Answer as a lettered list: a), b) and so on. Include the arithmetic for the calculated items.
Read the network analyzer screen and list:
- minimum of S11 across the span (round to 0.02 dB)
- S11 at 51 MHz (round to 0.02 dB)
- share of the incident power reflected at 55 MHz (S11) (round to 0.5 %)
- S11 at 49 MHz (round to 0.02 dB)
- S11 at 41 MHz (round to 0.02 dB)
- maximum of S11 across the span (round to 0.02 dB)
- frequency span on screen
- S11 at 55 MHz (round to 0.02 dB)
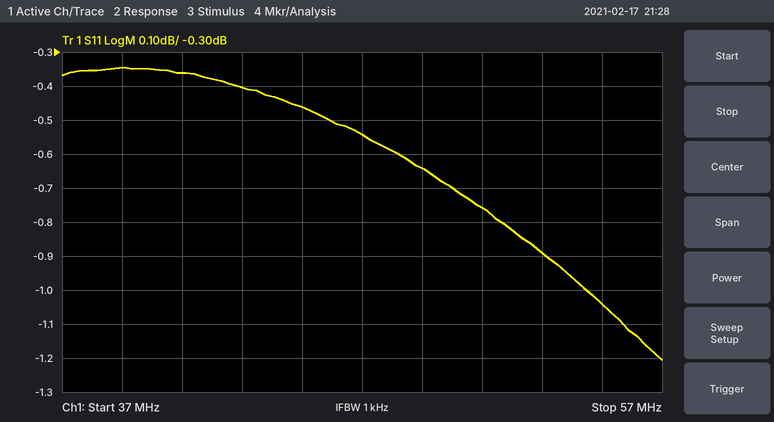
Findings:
a) -1.20 dB
b) -0.76 dB
c) 10^(-1.04/10) ≈ 78.7 %, so 78.5 % to the nearest 0.5 %
d) -0.64 dB
e) -0.36 dB
f) -0.34 dB
g) 20 MHz
h) -1.04 dB
